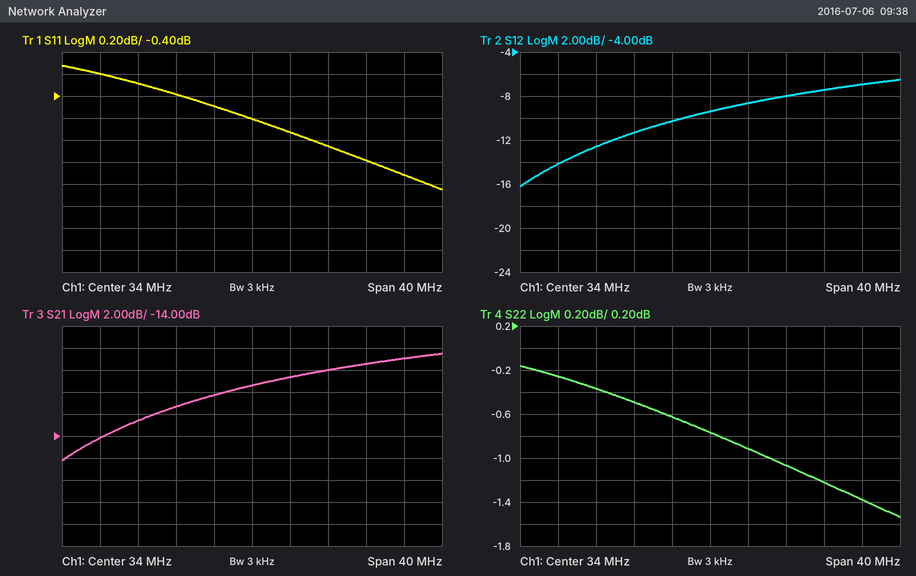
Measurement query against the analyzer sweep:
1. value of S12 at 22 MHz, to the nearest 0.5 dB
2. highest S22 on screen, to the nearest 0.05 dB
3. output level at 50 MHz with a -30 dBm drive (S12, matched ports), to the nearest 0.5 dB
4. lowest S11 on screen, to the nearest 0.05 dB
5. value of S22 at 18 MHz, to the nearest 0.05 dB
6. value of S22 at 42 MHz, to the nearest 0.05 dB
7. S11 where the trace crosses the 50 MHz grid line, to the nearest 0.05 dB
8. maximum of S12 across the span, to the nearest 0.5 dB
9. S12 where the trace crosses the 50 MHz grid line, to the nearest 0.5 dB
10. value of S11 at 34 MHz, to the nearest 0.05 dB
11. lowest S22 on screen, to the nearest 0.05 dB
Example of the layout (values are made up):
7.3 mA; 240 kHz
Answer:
-12.5 dB; -0.15 dB; -37.0 dBm; -1.25 dB; -0.25 dB; -1.05 dB; -1.10 dB; -6.5 dB; -7.0 dB; -0.60 dB; -1.55 dB
